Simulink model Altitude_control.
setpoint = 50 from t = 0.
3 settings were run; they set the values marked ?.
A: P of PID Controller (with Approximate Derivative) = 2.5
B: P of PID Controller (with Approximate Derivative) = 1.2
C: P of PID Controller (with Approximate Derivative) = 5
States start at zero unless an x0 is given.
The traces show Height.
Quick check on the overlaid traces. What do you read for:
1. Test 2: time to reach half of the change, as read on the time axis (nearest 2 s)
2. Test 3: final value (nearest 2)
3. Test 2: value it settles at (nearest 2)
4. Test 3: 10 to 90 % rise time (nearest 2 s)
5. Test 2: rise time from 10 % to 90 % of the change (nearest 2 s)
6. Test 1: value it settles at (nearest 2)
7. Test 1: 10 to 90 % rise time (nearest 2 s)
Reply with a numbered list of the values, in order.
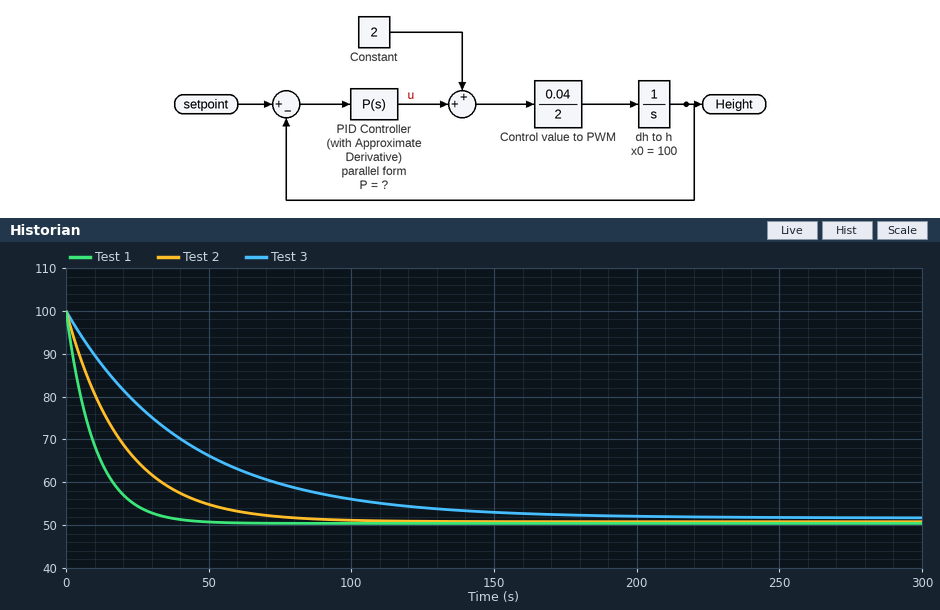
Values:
1. 14 s
2. 52
3. 50
4. 92 s
5. 44 s
6. 50
7. 22 s
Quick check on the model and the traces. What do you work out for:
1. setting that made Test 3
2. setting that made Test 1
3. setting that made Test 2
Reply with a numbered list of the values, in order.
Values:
1. B
2. C
3. A
